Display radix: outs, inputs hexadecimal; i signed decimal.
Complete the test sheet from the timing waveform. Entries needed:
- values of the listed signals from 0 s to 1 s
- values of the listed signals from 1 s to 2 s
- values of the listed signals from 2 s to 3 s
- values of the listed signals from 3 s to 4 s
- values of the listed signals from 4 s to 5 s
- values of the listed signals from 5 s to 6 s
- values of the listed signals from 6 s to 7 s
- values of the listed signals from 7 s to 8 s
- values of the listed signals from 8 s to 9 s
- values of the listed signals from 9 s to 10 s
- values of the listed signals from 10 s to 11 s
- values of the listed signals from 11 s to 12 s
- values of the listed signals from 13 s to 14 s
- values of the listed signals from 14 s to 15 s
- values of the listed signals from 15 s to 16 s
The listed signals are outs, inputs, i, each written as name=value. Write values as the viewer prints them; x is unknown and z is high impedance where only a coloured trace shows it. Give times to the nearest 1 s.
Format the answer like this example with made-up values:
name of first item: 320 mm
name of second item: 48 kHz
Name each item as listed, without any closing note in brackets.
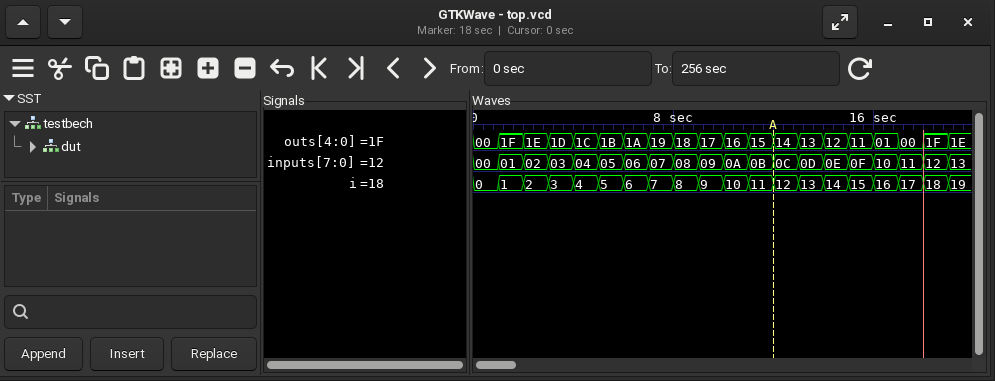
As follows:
values of the listed signals from 0 s to 1 s: outs=00, inputs=00, i=0
values of the listed signals from 1 s to 2 s: outs=1F, inputs=01, i=1
values of the listed signals from 2 s to 3 s: outs=1E, inputs=02, i=2
values of the listed signals from 3 s to 4 s: outs=1D, inputs=03, i=3
values of the listed signals from 4 s to 5 s: outs=1C, inputs=04, i=4
values of the listed signals from 5 s to 6 s: outs=1B, inputs=05, i=5
values of the listed signals from 6 s to 7 s: outs=1A, inputs=06, i=6
values of the listed signals from 7 s to 8 s: outs=19, inputs=07, i=7
values of the listed signals from 8 s to 9 s: outs=18, inputs=08, i=8
values of the listed signals from 9 s to 10 s: outs=17, inputs=09, i=9
values of the listed signals from 10 s to 11 s: outs=16, inputs=0A, i=10
values of the listed signals from 11 s to 12 s: outs=15, inputs=0B, i=11
values of the listed signals from 13 s to 14 s: outs=13, inputs=0D, i=13
values of the listed signals from 14 s to 15 s: outs=12, inputs=0E, i=14
values of the listed signals from 15 s to 16 s: outs=11, inputs=0F, i=15
